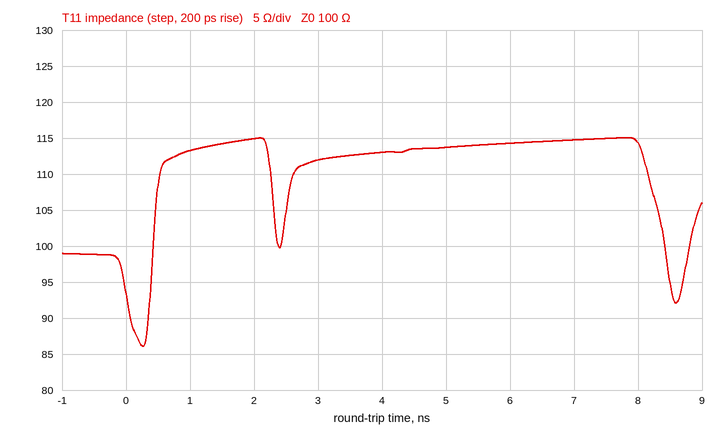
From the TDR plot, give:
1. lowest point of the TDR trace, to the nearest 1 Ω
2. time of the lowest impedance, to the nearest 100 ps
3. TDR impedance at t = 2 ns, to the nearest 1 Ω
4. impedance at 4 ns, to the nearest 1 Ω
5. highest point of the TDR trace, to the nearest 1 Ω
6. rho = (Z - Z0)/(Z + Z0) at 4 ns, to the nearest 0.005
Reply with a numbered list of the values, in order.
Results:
1. 86 Ω
2. 300 ps
3. 115 Ω
4. 113 Ω
5. 115 Ω
6. +0.060
